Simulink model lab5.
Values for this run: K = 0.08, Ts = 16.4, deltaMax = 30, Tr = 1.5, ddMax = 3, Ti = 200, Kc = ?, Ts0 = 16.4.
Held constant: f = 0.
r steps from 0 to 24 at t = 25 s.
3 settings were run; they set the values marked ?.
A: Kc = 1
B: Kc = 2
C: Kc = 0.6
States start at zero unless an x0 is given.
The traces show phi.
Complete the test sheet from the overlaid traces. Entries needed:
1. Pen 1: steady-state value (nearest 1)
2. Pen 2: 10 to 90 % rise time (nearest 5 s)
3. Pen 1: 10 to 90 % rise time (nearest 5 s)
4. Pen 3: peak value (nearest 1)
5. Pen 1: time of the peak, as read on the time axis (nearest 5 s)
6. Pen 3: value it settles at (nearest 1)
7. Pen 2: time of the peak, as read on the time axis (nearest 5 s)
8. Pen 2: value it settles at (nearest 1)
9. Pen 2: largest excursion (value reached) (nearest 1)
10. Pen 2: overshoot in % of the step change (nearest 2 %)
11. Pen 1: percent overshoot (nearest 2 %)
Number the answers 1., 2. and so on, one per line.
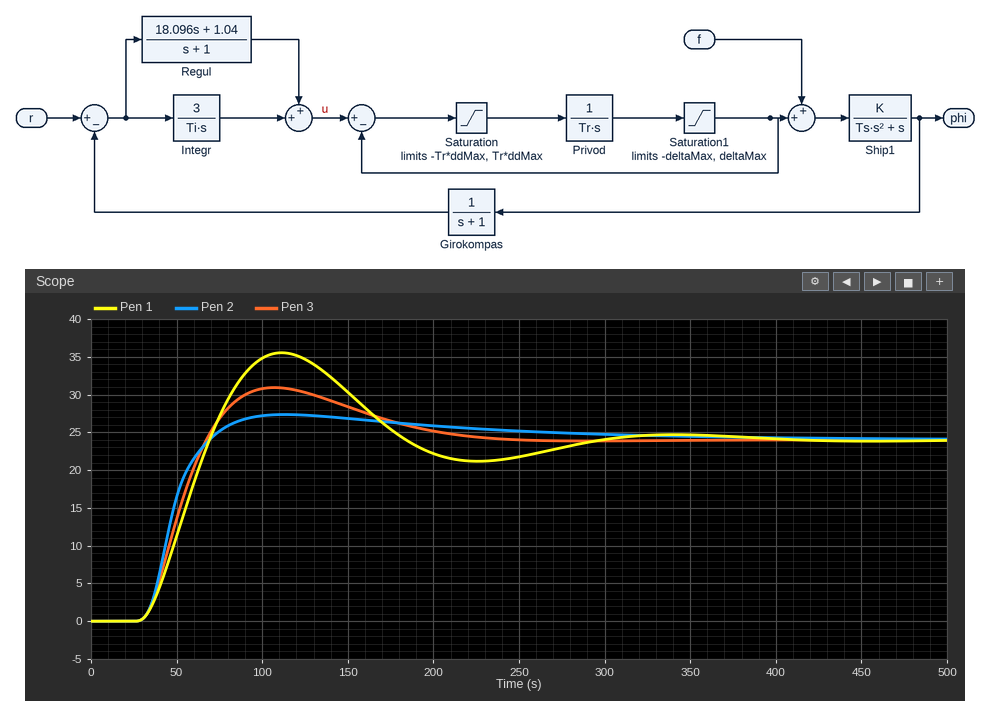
1. 24
2. 25 s
3. 30 s
4. 31
5. 110 s
6. 24
7. 115 s
8. 24
9. 27
10. 14 %
11. 48 %
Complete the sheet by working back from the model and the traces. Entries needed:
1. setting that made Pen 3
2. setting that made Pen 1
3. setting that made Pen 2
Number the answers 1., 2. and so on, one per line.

1. A
2. C
3. B
